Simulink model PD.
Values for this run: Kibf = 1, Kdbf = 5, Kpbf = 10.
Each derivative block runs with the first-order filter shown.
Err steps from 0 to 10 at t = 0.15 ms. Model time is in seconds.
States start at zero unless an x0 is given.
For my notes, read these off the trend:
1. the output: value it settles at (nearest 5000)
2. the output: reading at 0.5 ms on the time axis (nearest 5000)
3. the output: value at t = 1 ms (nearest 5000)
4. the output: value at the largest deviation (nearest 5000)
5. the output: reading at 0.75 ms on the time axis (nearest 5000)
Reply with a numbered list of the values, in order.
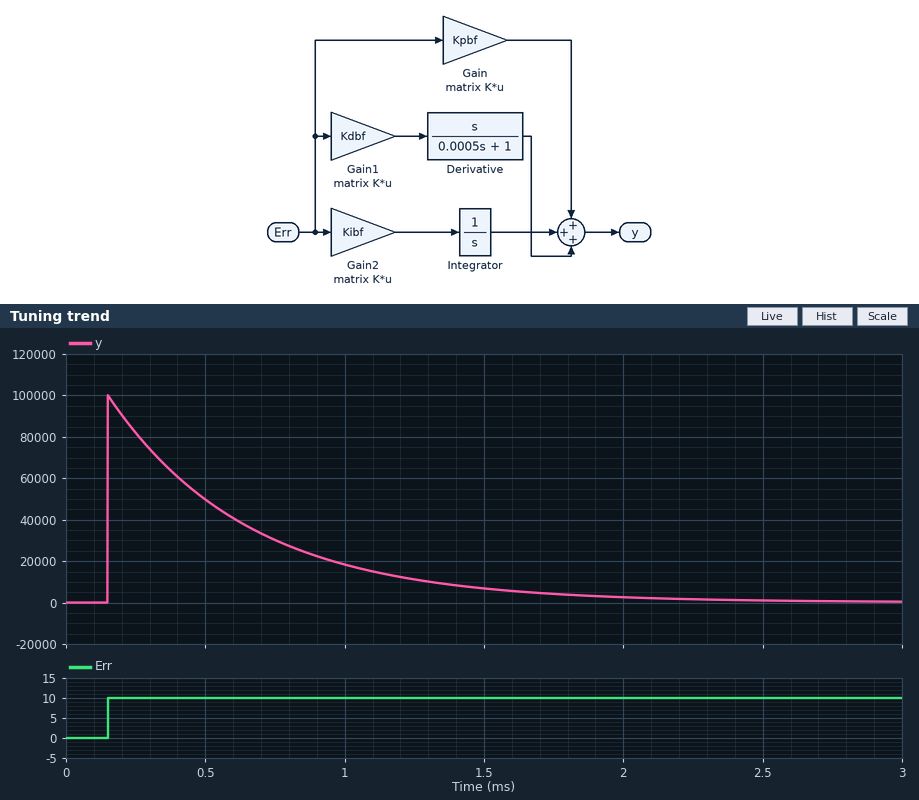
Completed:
1. 0
2. 50000
3. 20000
4. 100000
5. 30000
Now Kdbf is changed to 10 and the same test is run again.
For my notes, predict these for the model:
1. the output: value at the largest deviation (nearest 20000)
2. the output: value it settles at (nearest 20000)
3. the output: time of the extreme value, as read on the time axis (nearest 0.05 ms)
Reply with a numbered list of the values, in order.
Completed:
1. 200000
2. 0
3. 0.15 ms
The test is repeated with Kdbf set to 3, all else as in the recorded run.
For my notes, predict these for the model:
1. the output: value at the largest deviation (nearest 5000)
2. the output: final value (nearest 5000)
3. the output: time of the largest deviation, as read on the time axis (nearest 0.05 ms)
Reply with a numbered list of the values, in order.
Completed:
1. 60000
2. 0
3. 0.15 ms
